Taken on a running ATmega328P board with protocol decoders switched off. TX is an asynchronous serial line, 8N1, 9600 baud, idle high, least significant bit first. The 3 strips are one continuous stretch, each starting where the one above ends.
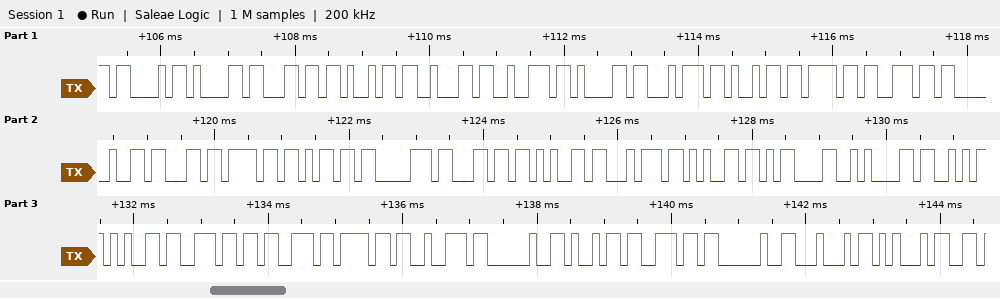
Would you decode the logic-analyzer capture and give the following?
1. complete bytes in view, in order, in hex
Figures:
43 61 6C 69 62 72 61 74 69 6F 6E 20 63 6F 6D 70 6C 65 74 65 0D 0A 53 65 6E 73 6F 72 20 69 6E 20 44 45
